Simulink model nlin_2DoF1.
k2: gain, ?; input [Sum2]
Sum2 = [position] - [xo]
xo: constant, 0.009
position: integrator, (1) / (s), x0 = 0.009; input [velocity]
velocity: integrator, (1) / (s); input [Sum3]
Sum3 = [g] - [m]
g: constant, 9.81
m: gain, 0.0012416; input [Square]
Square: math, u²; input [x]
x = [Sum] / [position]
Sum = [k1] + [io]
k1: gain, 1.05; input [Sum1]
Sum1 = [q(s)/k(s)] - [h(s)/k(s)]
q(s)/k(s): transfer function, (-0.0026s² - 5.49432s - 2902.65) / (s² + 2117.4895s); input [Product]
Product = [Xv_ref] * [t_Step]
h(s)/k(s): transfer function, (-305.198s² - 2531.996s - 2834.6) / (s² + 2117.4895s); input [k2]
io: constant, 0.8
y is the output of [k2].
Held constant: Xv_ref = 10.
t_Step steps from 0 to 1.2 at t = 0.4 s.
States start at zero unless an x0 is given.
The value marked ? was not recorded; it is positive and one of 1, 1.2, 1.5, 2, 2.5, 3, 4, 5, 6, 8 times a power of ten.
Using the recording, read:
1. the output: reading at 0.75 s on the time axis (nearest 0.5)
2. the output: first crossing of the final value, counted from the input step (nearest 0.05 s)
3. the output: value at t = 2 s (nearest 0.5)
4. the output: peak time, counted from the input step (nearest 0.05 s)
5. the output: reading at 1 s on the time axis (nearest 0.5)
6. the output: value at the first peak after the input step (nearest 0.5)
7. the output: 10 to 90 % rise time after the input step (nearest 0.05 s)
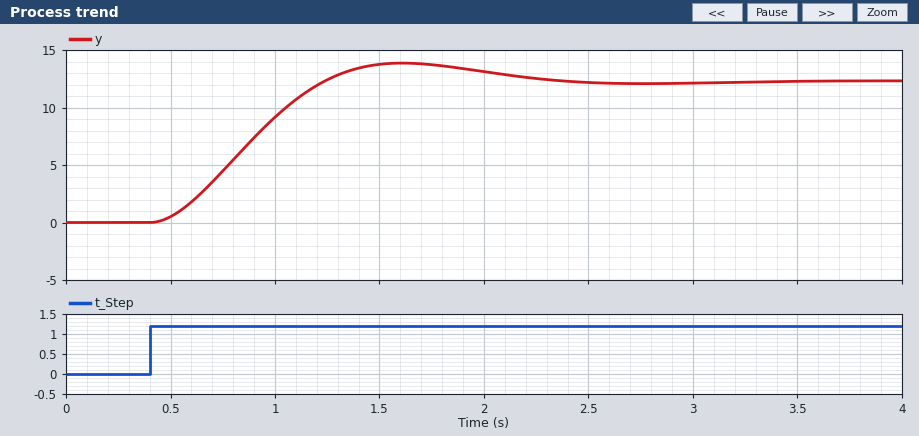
4.5
0.85 s
13.0
1.20 s
9.0
14.0
0.55 s
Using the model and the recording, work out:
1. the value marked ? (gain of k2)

120
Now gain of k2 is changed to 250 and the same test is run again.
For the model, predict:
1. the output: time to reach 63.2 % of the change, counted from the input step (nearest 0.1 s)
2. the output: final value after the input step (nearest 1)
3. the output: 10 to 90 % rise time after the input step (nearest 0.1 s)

0.7 s
12
1.1 s
